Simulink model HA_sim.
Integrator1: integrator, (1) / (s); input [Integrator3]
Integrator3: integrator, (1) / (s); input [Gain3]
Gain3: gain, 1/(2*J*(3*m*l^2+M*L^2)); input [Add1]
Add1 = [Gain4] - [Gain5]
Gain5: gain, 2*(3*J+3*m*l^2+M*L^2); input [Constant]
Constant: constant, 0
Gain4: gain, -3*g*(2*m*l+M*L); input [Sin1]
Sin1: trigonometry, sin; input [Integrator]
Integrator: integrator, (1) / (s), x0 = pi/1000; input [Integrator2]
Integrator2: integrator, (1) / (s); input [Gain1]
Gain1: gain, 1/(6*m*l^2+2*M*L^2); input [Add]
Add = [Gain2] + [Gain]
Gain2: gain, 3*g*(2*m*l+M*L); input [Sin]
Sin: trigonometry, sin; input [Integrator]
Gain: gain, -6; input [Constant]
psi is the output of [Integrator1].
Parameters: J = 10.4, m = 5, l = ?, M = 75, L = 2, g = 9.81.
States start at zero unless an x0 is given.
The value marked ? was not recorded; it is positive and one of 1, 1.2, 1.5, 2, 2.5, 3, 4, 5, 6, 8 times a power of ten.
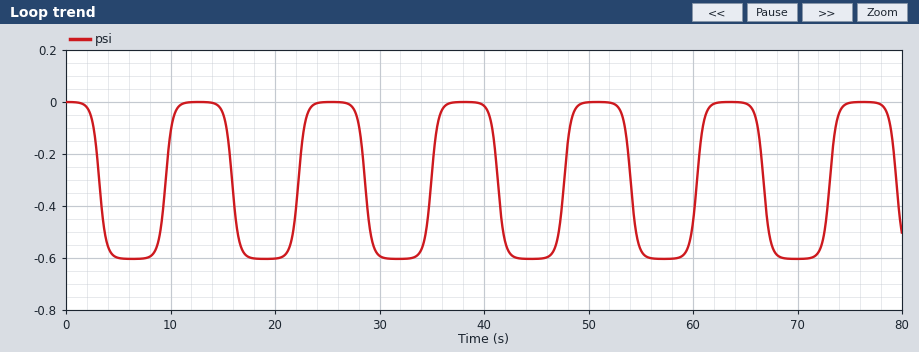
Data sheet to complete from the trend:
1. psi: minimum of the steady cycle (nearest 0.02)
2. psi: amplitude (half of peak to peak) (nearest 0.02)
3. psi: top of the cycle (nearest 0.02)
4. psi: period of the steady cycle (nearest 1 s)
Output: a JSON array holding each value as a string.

["-0.60", "0.30", "0.00", "13 s"]
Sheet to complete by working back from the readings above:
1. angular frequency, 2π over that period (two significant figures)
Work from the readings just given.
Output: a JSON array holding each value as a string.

["0.48 rad/s"]
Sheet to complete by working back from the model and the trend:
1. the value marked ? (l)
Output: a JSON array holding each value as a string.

["3"]
